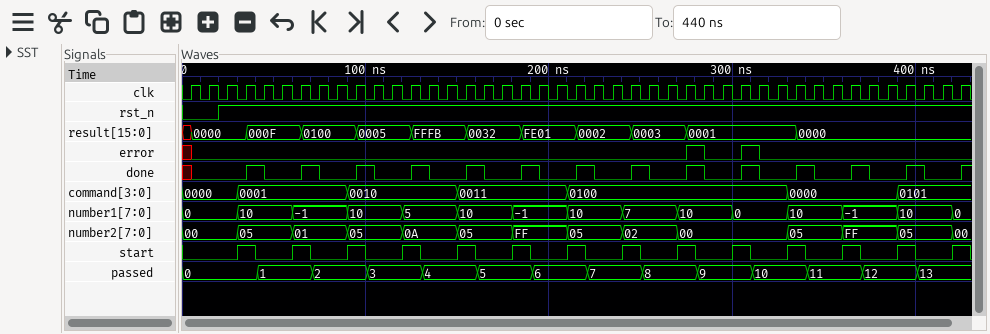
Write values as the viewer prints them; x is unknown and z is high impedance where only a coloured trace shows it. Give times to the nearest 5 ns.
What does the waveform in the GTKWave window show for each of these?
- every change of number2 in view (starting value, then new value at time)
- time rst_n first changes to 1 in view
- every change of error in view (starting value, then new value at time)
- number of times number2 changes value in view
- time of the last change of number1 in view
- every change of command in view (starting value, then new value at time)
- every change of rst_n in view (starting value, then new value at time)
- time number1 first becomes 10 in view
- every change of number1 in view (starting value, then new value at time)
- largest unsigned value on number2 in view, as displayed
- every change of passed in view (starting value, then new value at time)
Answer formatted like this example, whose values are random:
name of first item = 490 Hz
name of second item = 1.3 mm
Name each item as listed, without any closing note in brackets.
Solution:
every change of number2 in view = 00, 05 at 30 ns, 01 at 60 ns, 05 at 90 ns, 0A at 120 ns, 05 at 150 ns, FF at 180 ns, 05 at 210 ns, 02 at 240 ns, 00 at 270 ns, 05 at 330 ns, FF at 360 ns, 05 at 390 ns, 00 at 420 ns
time rst_n first changes to 1 in view = 20 ns
every change of error in view = x, 0 at 5 ns, 1 at 275 ns, 0 at 285 ns, 1 at 305 ns, 0 at 315 ns
number of times number2 changes value in view = 13
time of the last change of number1 in view = 420 ns
every change of command in view = 0000, 0001 at 30 ns, 0010 at 90 ns, 0011 at 150 ns, 0100 at 210 ns, 0000 at 330 ns, 0101 at 390 ns
every change of rst_n in view = 0, 1 at 20 ns
time number1 first becomes 10 in view = 30 ns
every change of number1 in view = 0, 10 at 30 ns, -1 at 60 ns, 10 at 90 ns, 5 at 120 ns, 10 at 150 ns, -1 at 180 ns, 10 at 210 ns, 7 at 240 ns, 10 at 270 ns, 0 at 300 ns, 10 at 330 ns, -1 at 360 ns, 10 at 390 ns, 0 at 420 ns
largest unsigned value on number2 in view, as displayed = FF
every change of passed in view = 0, 1 at 40 ns, 2 at 70 ns, 3 at 100 ns, 4 at 130 ns, 5 at 160 ns, 6 at 190 ns, 7 at 220 ns, 8 at 250 ns, 9 at 280 ns, 10 at 310 ns, 11 at 340 ns, 12 at 370 ns, 13 at 400 ns
